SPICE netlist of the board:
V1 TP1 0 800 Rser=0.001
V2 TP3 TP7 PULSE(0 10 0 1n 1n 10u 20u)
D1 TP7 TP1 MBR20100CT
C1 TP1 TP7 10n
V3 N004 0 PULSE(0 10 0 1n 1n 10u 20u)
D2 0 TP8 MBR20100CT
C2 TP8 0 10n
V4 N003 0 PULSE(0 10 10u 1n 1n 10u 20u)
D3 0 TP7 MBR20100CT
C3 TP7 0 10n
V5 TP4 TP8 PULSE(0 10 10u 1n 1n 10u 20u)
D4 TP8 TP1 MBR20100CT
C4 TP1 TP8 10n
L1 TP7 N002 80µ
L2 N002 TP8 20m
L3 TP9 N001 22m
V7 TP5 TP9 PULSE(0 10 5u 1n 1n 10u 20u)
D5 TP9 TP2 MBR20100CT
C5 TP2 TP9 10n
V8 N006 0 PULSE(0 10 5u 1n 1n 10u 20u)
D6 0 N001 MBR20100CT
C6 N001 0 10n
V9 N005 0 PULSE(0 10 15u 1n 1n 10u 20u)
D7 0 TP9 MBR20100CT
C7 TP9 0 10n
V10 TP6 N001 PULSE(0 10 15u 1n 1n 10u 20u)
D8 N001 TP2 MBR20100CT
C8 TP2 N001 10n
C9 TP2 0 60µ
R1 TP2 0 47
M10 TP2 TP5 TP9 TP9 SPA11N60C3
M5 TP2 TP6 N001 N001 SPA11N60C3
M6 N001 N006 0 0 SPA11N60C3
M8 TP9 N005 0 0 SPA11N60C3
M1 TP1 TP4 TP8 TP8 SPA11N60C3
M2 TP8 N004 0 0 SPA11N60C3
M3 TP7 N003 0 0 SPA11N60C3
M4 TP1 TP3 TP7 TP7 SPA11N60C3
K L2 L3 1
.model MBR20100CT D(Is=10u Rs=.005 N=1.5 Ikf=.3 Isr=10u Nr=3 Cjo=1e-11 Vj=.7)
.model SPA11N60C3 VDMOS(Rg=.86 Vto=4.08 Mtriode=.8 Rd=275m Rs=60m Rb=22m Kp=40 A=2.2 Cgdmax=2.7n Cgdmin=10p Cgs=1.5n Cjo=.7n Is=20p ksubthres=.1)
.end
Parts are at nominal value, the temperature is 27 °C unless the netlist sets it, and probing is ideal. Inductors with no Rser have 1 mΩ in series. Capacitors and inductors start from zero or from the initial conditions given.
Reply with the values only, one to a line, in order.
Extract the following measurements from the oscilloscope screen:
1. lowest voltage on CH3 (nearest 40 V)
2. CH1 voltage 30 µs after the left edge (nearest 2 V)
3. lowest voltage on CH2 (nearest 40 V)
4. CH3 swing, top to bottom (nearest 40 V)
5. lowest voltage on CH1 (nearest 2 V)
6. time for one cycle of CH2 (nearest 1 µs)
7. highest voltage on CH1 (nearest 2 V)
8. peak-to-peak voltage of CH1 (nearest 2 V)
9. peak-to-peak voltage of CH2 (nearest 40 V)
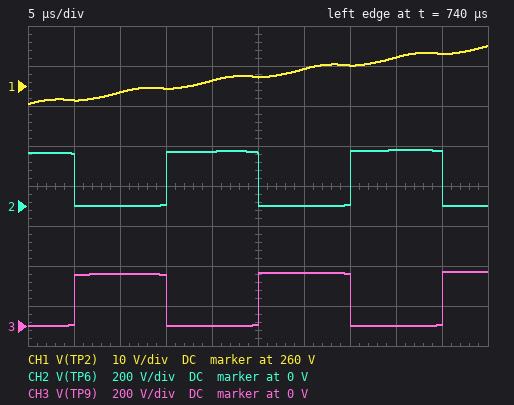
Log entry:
0 V
264 V
0 V
280 V
256 V
20 µs
270 V
14 V
280 V
